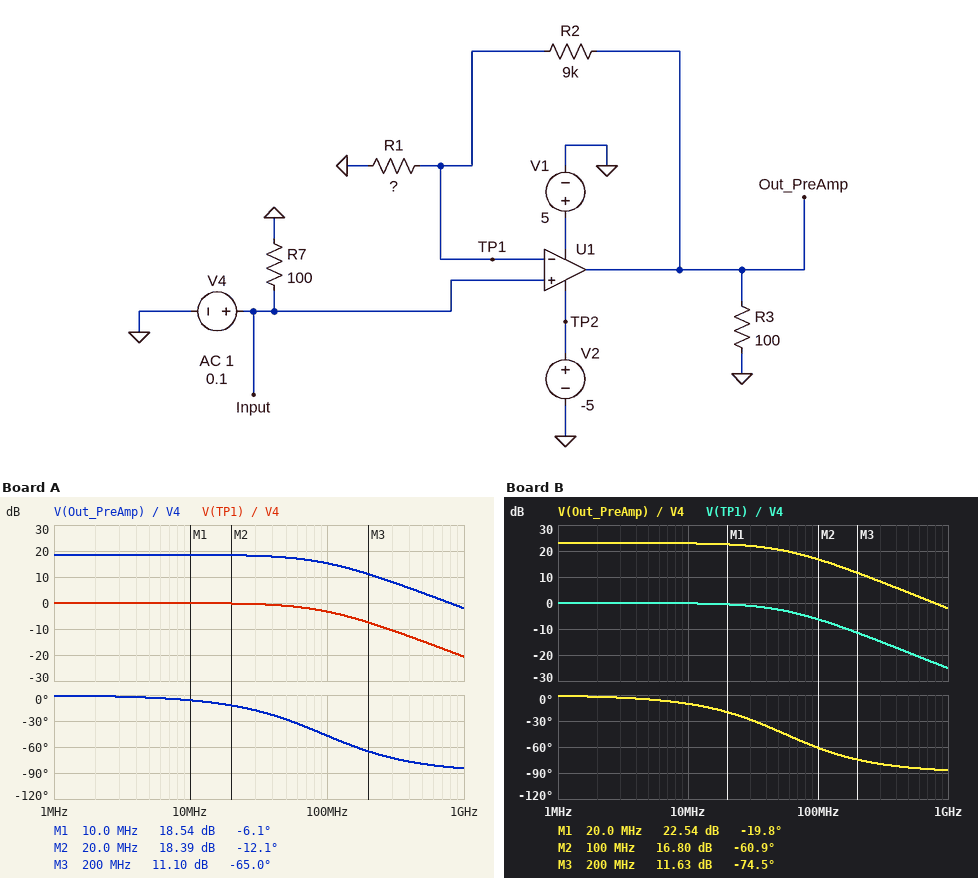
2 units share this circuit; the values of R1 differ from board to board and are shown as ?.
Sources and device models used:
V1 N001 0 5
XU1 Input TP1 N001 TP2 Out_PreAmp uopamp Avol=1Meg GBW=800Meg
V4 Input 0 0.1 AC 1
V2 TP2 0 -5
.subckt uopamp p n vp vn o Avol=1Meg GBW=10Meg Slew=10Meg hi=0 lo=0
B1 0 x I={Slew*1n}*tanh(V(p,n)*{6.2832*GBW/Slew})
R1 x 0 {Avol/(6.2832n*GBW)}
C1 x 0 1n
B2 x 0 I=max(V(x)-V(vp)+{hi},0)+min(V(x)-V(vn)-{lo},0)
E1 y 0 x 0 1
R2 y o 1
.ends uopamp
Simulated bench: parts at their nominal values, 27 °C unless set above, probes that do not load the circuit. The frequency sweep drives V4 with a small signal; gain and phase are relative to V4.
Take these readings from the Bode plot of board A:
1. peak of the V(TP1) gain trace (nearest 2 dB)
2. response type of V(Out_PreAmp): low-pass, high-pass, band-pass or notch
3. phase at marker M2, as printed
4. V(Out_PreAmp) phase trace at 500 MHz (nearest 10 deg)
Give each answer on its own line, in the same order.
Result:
0 dB
low-pass
-12.1 deg
-80 deg
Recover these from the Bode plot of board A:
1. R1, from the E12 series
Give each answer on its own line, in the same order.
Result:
1.2 kΩ
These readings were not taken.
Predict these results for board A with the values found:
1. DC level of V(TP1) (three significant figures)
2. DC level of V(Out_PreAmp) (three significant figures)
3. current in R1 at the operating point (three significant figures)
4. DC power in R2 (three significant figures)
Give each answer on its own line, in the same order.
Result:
100 mV
850 mV
83.3 µA
62.5 µW
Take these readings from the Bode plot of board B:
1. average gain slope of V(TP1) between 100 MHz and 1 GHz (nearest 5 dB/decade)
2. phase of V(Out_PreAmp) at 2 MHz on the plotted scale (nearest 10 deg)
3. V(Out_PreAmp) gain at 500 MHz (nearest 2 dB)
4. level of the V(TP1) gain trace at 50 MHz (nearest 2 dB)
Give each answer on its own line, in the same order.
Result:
-20 dB/decade
0 deg
4 dB
-2 dB
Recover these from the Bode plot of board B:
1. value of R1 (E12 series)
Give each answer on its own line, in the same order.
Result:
680 Ω
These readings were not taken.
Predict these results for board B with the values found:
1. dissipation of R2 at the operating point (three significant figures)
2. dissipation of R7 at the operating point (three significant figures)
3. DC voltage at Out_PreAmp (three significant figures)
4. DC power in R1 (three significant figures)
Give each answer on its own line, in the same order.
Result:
195 µW
100 µW
1.42 V
14.7 µW
